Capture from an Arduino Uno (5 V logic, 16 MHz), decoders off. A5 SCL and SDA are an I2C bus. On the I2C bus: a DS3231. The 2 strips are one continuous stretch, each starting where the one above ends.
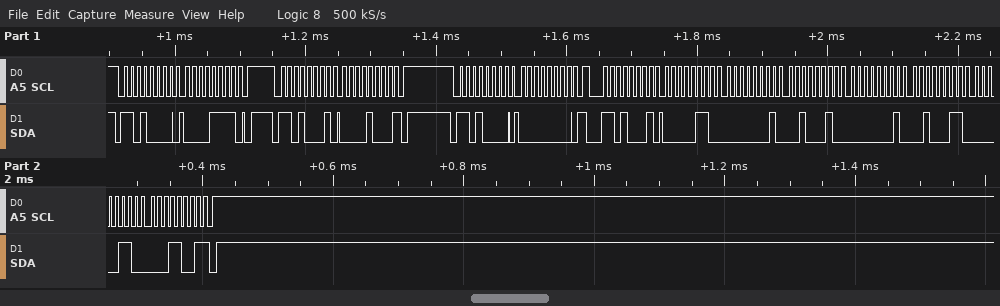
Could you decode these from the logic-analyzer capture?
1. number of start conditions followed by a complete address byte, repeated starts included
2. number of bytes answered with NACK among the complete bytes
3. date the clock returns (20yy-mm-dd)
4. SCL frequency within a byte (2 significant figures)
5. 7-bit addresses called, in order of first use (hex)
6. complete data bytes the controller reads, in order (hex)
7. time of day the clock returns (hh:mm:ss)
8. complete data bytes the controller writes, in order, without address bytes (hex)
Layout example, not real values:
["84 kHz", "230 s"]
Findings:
["4", "2", "2019-06-23", "100 kHz", "0x68", "08 06 01 22 01 23 06 19", "22:01:06", "0F 00"]
